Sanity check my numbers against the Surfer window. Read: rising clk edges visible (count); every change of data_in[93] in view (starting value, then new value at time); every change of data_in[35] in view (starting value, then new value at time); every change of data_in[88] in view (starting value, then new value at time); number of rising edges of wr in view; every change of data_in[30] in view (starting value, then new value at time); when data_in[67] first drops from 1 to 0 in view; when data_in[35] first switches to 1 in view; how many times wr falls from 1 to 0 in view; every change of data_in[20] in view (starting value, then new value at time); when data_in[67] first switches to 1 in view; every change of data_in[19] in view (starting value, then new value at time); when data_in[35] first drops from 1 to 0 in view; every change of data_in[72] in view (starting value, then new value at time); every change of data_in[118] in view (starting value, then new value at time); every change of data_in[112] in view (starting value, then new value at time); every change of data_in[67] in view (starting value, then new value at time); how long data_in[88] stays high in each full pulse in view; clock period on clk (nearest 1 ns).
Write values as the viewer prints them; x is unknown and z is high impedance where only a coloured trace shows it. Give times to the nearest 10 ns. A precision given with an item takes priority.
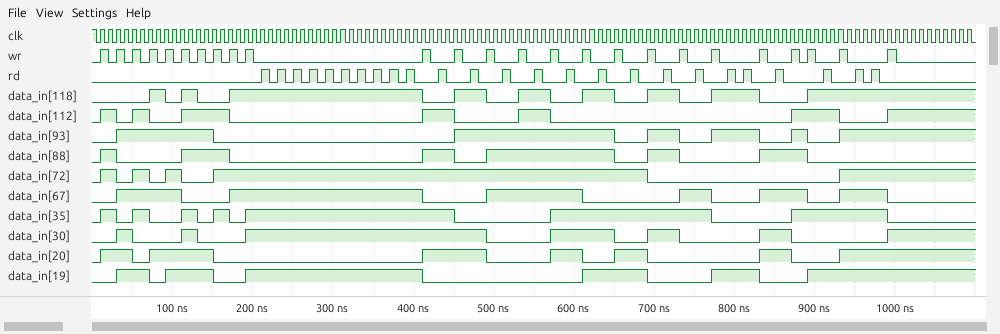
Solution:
109
0, 1 at 30 ns, 0 at 150 ns, 1 at 450 ns, 0 at 650 ns, 1 at 690 ns, 0 at 730 ns, 1 at 770 ns, 0 at 830 ns, 1 at 870 ns, 0 at 890 ns, 1 at 930 ns
0, 1 at 10 ns, 0 at 30 ns, 1 at 50 ns, 0 at 70 ns, 1 at 110 ns, 0 at 130 ns, 1 at 150 ns, 0 at 170 ns, 1 at 190 ns, 0 at 450 ns, 1 at 570 ns, 0 at 770 ns, 1 at 870 ns, 0 at 990 ns
0, 1 at 10 ns, 0 at 30 ns, 1 at 110 ns, 0 at 170 ns, 1 at 410 ns, 0 at 450 ns, 1 at 490 ns, 0 at 650 ns, 1 at 690 ns, 0 at 730 ns, 1 at 830 ns, 0 at 890 ns
25
0, 1 at 30 ns, 0 at 50 ns, 1 at 110 ns, 0 at 130 ns, 1 at 190 ns, 0 at 490 ns, 1 at 570 ns, 0 at 650 ns, 1 at 690 ns, 0 at 730 ns, 1 at 830 ns, 0 at 870 ns, 1 at 990 ns
110 ns
10 ns
25
0, 1 at 10 ns, 0 at 50 ns, 1 at 70 ns, 0 at 150 ns, 1 at 410 ns, 0 at 490 ns, 1 at 570 ns, 0 at 610 ns, 1 at 650 ns, 0 at 690 ns, 1 at 830 ns, 0 at 870 ns, 1 at 930 ns
30 ns
0, 1 at 30 ns, 0 at 70 ns, 1 at 90 ns, 0 at 150 ns, 1 at 190 ns, 0 at 410 ns, 1 at 610 ns, 0 at 690 ns, 1 at 770 ns, 0 at 830 ns, 1 at 890 ns
30 ns
0, 1 at 10 ns, 0 at 30 ns, 1 at 50 ns, 0 at 70 ns, 1 at 90 ns, 0 at 110 ns, 1 at 150 ns, 0 at 690 ns, 1 at 930 ns
0, 1 at 70 ns, 0 at 90 ns, 1 at 110 ns, 0 at 130 ns, 1 at 170 ns, 0 at 410 ns, 1 at 450 ns, 0 at 490 ns, 1 at 530 ns, 0 at 570 ns, 1 at 610 ns, 0 at 650 ns, 1 at 690 ns, 0 at 730 ns, 1 at 770 ns, 0 at 830 ns, 1 at 890 ns
0, 1 at 10 ns, 0 at 30 ns, 1 at 50 ns, 0 at 70 ns, 1 at 110 ns, 0 at 170 ns, 1 at 410 ns, 0 at 450 ns, 1 at 530 ns, 0 at 570 ns, 1 at 870 ns, 0 at 930 ns, 1 at 990 ns
0, 1 at 30 ns, 0 at 110 ns, 1 at 170 ns, 0 at 410 ns, 1 at 490 ns, 0 at 610 ns, 1 at 730 ns, 0 at 770 ns, 1 at 830 ns, 0 at 890 ns, 1 at 930 ns, 0 at 990 ns
20 ns, 60 ns, 40 ns, 160 ns, 40 ns, 60 ns
10 ns
